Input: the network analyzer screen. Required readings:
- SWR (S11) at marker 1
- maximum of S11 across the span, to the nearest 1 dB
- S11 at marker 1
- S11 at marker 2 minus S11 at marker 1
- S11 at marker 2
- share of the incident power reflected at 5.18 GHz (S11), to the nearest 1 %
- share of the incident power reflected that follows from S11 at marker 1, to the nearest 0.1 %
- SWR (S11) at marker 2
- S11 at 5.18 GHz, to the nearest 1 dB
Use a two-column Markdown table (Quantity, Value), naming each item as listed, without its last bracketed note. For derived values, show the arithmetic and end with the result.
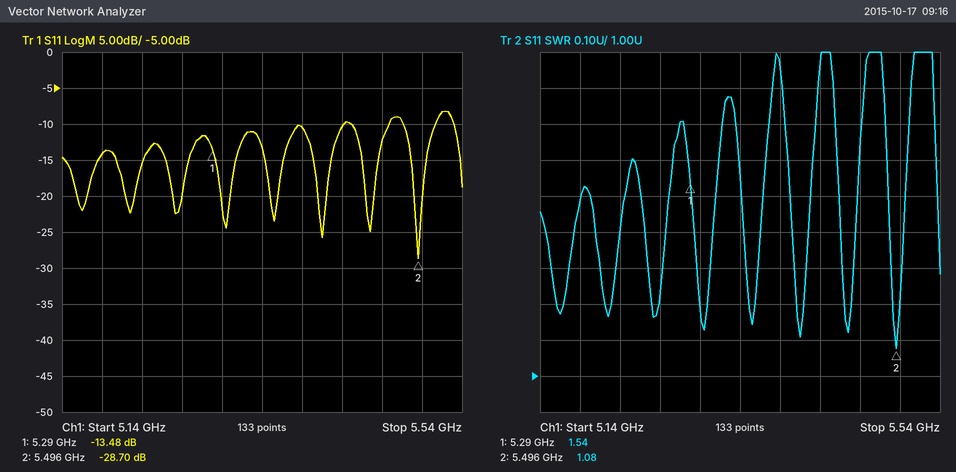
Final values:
| Quantity | Value |
|---|---|
| SWR (S11) at marker 1 | 1.54 |
| maximum of S11 across the span, to the nearest 1 dB | -8 dB |
| S11 at marker 1 | -13.48 dB |
| S11 at marker 2 minus S11 at marker 1 | -28.7 − (-13.48) = -15.22 dB |
| S11 at marker 2 | -28.70 dB |
| share of the incident power reflected at 5.18 GHz (S11), to the nearest 1 % | 10^(-14/10) ≈ 4 % |
| share of the incident power reflected that follows from S11 at marker 1, to the nearest 0.1 % | 10^(-13.48/10) ≈ 4.5 % |
| SWR (S11) at marker 2 | 1.08 |
| S11 at 5.18 GHz, to the nearest 1 dB | -14 dB |
